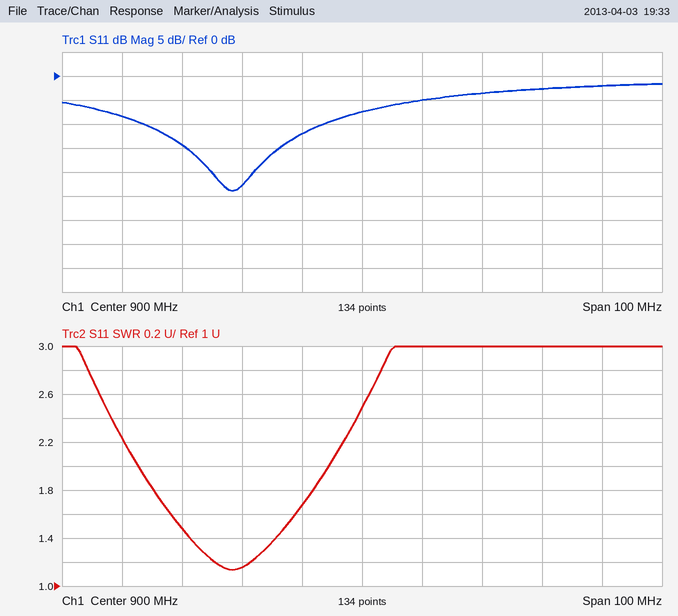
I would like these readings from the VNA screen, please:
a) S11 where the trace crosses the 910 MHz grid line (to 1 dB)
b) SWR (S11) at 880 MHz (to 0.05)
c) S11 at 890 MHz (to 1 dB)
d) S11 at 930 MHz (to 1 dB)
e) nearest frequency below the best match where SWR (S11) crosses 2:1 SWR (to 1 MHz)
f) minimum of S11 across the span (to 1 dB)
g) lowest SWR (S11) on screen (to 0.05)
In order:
-5 dB
1.15
-12 dB
-3 dB
863 MHz
-24 dB
1.15
